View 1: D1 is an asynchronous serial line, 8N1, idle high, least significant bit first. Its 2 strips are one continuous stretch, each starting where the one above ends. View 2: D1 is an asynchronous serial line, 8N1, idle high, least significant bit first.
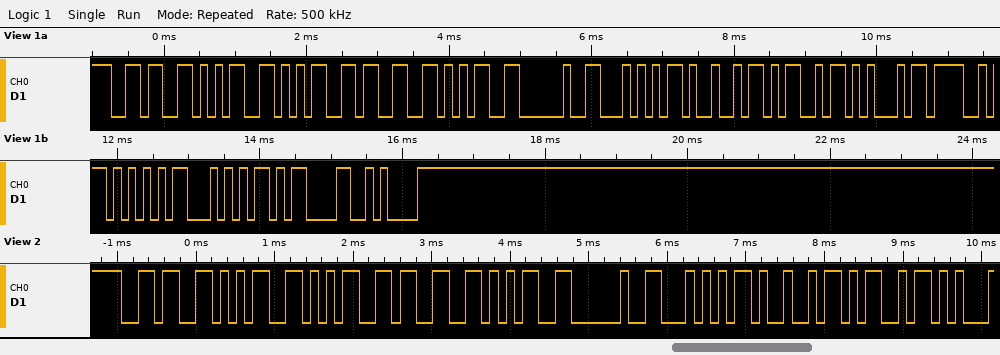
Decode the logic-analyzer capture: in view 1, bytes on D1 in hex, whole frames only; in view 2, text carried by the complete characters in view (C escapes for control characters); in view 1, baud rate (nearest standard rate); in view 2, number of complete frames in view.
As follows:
0x36 0x35 0x35 0x33 0x35 0x20 0x54 0x49 0x4D 0x45 0x4F 0x55 0x54 0x0D 0x0A
"65535 TIM"
9600 baud
9
